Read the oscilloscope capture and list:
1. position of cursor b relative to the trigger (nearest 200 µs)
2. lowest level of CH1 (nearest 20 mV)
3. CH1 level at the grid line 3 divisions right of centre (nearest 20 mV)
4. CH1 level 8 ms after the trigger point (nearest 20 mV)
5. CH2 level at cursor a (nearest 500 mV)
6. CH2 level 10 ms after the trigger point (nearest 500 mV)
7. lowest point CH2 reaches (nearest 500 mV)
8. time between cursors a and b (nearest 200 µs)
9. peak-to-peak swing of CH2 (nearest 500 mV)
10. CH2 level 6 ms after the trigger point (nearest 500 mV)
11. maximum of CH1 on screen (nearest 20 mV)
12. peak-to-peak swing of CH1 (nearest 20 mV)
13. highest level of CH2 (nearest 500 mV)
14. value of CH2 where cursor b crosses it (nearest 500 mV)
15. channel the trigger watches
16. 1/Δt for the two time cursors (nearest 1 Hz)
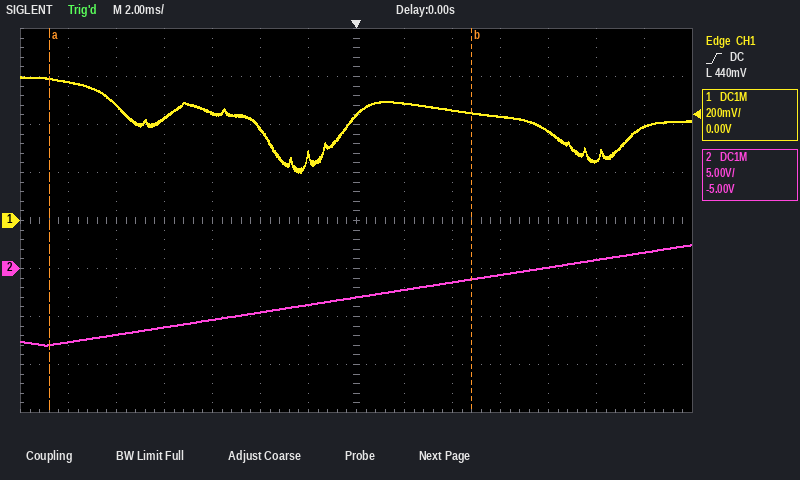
+4.8 ms
200 mV
440 mV
380 mV
-8.0 V
1.0 V
-8.0 V
17.6 ms
10.5 V
-500 mV
600 mV
400 mV
2.5 V
-1.0 V
CH1
57 Hz
